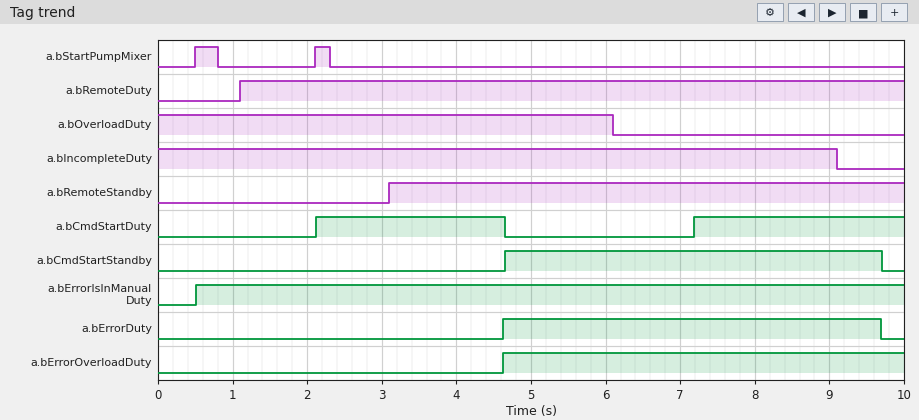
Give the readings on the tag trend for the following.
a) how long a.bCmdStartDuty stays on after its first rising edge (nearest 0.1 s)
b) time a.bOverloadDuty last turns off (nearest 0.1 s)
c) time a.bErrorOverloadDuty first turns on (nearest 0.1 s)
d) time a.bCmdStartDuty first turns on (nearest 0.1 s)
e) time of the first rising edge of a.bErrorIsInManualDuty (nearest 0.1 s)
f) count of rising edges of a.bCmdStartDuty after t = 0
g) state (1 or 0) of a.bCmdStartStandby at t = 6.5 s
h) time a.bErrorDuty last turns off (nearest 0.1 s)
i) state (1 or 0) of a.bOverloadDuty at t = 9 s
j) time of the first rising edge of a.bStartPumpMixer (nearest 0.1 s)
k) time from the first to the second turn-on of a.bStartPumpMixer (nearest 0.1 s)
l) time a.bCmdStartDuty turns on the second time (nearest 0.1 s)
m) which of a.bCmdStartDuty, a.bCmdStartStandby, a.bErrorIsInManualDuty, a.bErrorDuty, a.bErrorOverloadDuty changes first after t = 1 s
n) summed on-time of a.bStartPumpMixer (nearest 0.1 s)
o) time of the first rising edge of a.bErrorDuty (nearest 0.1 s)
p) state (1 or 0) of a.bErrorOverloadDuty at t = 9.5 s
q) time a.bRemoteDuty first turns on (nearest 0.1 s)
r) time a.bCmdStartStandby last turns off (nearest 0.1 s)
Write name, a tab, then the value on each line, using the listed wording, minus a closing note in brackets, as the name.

how long a.bCmdStartDuty stays on after its first rising edge	2.5 s
time a.bOverloadDuty last turns off	6.1 s
time a.bErrorOverloadDuty first turns on	4.6 s
time a.bCmdStartDuty first turns on	2.1 s
time of the first rising edge of a.bErrorIsInManualDuty	0.5 s
count of rising edges of a.bCmdStartDuty after t = 0	2
state (1 or 0) of a.bCmdStartStandby at t = 6.5 s	1
time a.bErrorDuty last turns off	9.7 s
state (1 or 0) of a.bOverloadDuty at t = 9 s	0
time of the first rising edge of a.bStartPumpMixer	0.5 s
time from the first to the second turn-on of a.bStartPumpMixer	1.6 s
time a.bCmdStartDuty turns on the second time	7.2 s
which of a.bCmdStartDuty, a.bCmdStartStandby, a.bErrorIsInManualDuty, a.bErrorDuty, a.bErrorOverloadDuty changes first after t = 1 s	a.bCmdStartDuty
summed on-time of a.bStartPumpMixer	0.5 s
time of the first rising edge of a.bErrorDuty	4.6 s
state (1 or 0) of a.bErrorOverloadDuty at t = 9.5 s	1
time a.bRemoteDuty first turns on	1.1 s
time a.bCmdStartStandby last turns off	9.7 s
